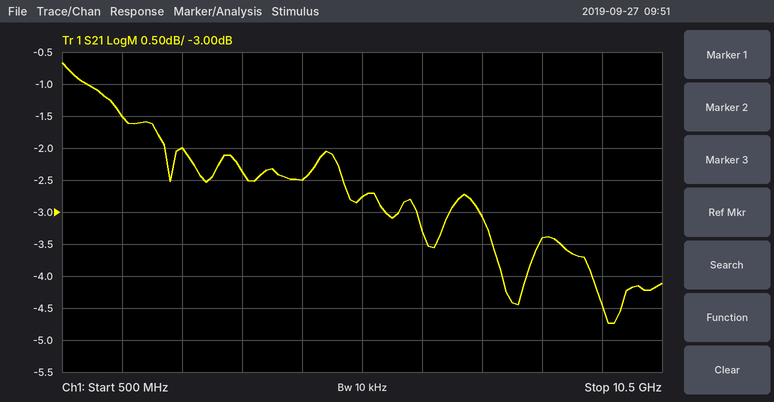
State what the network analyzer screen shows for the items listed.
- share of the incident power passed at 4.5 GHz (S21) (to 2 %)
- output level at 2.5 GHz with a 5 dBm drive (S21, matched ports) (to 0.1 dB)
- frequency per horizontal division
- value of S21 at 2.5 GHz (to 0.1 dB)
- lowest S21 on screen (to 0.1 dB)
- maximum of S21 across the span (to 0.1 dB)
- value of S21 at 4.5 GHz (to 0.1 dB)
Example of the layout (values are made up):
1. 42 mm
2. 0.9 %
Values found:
1. 56 %
2. 3.0 dBm
3. 1 GHz
4. -2.0 dB
5. -4.7 dB
6. -0.7 dB
7. -2.5 dB
